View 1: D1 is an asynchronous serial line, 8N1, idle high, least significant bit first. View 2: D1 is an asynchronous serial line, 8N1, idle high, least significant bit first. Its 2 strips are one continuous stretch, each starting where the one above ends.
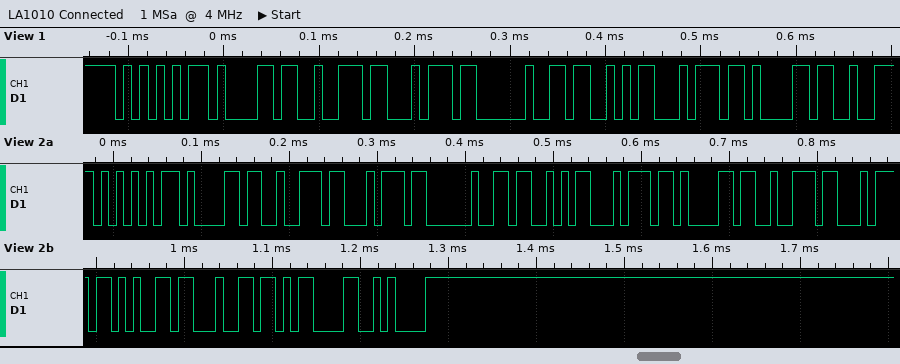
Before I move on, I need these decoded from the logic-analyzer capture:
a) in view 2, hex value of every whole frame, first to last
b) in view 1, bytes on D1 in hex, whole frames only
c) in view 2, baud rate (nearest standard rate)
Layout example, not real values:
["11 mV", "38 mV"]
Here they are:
["0x55 0x61 0x72 0x74 0x20 0x53 0x74 0x61 0x72 0x74 0x65 0x64 0x0D 0x0A", "55 61 72 74 20 53 74 61", "115200 baud"]
